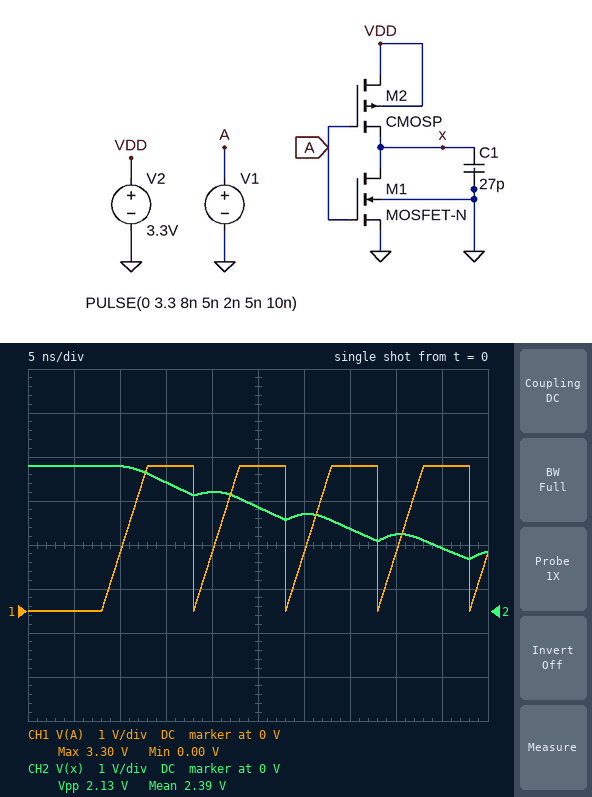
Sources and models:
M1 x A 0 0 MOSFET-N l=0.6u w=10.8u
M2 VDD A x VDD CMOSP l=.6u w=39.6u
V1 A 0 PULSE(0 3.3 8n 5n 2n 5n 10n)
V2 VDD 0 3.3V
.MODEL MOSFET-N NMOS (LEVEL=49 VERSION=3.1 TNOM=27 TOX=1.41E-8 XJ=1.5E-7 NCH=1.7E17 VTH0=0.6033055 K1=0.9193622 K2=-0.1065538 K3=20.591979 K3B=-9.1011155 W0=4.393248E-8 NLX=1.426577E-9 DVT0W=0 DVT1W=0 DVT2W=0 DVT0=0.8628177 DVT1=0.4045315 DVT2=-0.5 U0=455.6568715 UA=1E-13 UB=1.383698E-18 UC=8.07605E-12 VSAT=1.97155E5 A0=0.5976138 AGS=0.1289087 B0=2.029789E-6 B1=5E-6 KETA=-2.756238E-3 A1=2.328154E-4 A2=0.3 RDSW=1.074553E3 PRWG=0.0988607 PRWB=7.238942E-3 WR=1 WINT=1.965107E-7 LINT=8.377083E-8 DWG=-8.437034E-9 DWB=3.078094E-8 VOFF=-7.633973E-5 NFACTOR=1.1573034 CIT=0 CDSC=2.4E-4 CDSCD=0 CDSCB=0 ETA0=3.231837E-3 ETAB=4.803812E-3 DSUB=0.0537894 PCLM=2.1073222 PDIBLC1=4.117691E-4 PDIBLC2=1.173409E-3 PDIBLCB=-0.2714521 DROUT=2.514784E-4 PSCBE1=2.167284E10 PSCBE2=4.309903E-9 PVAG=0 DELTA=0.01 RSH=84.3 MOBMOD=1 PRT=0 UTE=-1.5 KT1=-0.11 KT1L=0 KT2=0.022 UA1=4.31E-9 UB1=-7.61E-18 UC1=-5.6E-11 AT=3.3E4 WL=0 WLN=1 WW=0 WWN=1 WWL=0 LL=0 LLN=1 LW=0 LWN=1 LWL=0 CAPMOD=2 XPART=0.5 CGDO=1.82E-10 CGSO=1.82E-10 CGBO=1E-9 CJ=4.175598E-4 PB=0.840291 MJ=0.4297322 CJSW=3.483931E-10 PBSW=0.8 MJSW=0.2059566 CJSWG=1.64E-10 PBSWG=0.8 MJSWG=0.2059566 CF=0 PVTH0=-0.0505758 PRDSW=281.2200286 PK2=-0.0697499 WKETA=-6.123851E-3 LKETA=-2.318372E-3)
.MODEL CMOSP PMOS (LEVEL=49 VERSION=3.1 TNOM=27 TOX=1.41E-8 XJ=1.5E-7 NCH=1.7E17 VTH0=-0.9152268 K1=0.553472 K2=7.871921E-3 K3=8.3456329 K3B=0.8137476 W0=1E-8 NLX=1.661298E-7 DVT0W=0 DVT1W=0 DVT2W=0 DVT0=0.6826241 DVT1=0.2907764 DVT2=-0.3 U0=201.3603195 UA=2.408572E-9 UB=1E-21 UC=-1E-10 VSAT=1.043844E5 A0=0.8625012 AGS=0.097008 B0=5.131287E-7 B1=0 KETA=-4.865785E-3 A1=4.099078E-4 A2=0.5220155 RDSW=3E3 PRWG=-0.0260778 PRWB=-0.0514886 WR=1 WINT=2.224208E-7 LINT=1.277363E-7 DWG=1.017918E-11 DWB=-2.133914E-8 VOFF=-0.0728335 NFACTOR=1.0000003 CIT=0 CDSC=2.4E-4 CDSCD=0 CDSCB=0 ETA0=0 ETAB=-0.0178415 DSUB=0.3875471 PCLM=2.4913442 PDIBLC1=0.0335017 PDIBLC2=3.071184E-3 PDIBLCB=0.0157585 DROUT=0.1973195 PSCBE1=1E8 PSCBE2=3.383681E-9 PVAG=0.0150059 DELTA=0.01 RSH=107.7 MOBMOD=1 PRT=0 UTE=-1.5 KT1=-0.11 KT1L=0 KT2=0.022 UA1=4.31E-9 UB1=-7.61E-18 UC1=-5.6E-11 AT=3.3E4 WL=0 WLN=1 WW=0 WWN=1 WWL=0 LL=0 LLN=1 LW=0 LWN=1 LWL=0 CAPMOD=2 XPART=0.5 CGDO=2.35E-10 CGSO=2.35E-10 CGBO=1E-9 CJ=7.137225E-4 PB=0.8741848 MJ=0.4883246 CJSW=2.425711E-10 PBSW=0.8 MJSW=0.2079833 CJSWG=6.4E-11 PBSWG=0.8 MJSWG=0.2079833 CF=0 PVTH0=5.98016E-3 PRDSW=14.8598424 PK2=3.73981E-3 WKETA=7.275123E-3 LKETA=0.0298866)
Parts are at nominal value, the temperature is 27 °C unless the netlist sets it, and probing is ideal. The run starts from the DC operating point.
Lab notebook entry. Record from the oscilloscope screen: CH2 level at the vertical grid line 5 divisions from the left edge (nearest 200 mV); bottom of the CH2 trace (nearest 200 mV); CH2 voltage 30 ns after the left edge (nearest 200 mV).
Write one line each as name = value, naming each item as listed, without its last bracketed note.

CH2 level at the vertical grid line 5 divisions from the left edge = 2.4 V
bottom of the CH2 trace = 1.2 V
CH2 voltage 30 ns after the left edge = 2.2 V
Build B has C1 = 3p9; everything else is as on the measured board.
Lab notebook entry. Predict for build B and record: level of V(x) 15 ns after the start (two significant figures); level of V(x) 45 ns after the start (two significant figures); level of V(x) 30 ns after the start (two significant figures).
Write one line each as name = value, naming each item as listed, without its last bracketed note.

level of V(x) 15 ns after the start = 930 mV
level of V(x) 45 ns after the start = 200 mV
level of V(x) 30 ns after the start = 1.3 V
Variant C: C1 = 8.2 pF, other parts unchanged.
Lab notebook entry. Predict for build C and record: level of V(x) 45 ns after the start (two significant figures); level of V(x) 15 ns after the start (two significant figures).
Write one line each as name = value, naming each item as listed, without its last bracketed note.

level of V(x) 45 ns after the start = 320 mV
level of V(x) 15 ns after the start = 2.1 V
